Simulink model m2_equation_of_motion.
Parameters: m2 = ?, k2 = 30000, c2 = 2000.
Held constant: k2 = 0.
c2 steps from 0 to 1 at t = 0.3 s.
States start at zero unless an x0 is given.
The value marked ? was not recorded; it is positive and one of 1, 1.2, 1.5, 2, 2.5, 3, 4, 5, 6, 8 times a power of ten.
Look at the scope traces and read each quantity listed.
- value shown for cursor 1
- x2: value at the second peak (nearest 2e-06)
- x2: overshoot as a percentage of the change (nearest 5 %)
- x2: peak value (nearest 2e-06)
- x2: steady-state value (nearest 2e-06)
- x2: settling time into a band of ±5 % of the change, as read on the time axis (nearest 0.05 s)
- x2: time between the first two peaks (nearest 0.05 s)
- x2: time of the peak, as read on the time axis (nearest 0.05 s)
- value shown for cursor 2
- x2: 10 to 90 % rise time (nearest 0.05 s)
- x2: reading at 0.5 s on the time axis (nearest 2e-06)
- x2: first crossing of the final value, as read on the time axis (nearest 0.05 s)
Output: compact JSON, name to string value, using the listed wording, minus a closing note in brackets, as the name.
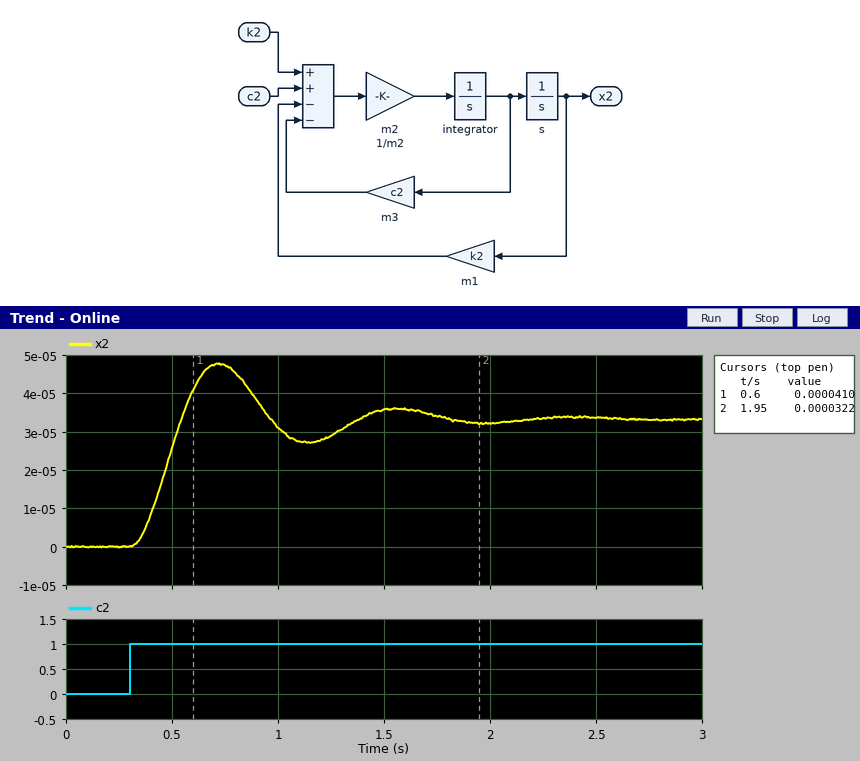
{"value shown for cursor 1": "0.0000410", "x2: value at the second peak": "0.000036", "x2: overshoot as a percentage of the change": "45 %", "x2: peak value": "0.000048", "x2: steady-state value": "0.000034", "x2: settling time into a band of ±5 % of the change, as read on the time axis": "1.70 s", "x2: time between the first two peaks": "0.85 s", "x2: time of the peak, as read on the time axis": "0.70 s", "value shown for cursor 2": "0.0000322", "x2: 10 to 90 % rise time": "0.15 s", "x2: reading at 0.5 s on the time axis": "0.000026", "x2: first crossing of the final value, as read on the time axis": "0.55 s"}
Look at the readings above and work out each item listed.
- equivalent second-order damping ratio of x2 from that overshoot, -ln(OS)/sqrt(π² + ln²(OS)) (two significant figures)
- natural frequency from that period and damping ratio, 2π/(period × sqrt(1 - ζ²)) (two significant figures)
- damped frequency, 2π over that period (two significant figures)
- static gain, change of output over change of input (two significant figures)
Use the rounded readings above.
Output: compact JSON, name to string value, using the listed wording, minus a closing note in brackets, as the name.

{"equivalent second-order damping ratio of x2 from that overshoot, -ln(OS)/sqrt(π² + ln²(OS))": "0.25", "natural frequency from that period and damping ratio, 2π/(period × sqrt(1 - ζ²))": "7.6 rad/s", "damped frequency, 2π over that period": "7.4 rad/s", "static gain, change of output over change of input": "0.000034"}
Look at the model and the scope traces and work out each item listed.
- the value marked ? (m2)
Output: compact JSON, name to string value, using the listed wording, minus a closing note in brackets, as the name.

{"the value marked ?": "500"}
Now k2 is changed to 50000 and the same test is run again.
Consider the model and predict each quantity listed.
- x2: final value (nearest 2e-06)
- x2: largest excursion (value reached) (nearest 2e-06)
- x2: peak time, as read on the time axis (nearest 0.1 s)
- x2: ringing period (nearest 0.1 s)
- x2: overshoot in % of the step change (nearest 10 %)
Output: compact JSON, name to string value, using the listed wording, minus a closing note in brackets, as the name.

{"x2: final value": "0.000020", "x2: largest excursion (value reached)": "0.000030", "x2: peak time, as read on the time axis": "0.6 s", "x2: ringing period": "0.6 s", "x2: overshoot in % of the step change": "50 %"}
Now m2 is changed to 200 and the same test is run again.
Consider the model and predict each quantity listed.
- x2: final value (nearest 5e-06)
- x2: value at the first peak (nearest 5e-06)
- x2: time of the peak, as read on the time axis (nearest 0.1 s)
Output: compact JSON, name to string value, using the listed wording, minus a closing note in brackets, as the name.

{"x2: final value": "0.000035", "x2: value at the first peak": "0.000040", "x2: time of the peak, as read on the time axis": "0.6 s"}
